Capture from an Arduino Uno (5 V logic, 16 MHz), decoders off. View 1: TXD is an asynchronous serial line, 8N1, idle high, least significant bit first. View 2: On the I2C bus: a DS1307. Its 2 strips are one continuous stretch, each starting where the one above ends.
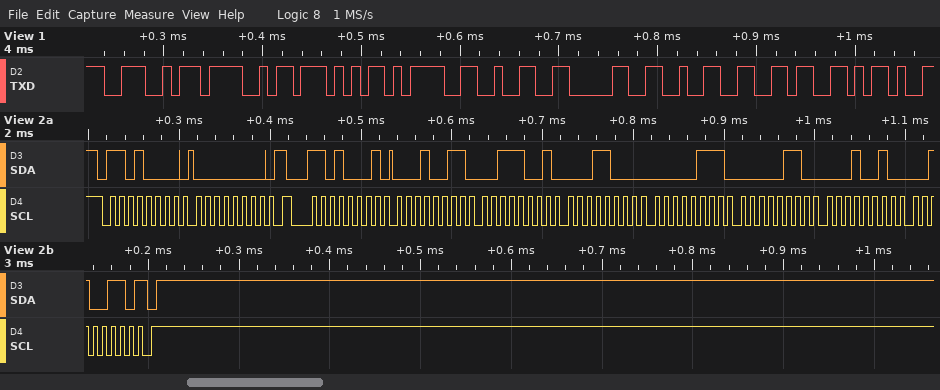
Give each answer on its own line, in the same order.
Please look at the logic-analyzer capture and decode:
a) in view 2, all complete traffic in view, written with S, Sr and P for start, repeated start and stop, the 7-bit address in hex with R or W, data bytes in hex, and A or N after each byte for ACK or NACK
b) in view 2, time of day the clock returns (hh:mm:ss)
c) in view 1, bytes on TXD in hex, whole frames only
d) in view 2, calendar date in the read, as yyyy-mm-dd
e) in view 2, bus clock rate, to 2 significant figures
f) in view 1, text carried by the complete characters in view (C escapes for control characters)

S 68W A 00 A Sr 68R A 13 A 39 A 18 A 07 A 06 A 12 A 26 N P
18:39:13
4E 4F 57 3D 32 30 32 36 2D
2026-12-06
100 kHz
"NOW=2026-"
